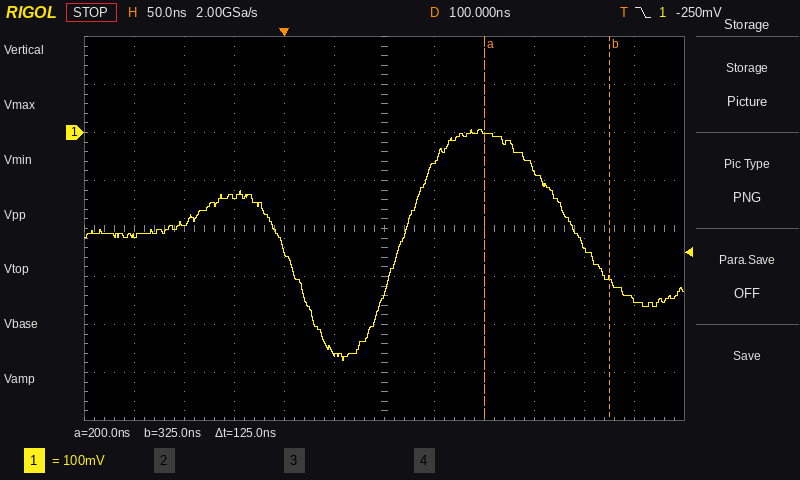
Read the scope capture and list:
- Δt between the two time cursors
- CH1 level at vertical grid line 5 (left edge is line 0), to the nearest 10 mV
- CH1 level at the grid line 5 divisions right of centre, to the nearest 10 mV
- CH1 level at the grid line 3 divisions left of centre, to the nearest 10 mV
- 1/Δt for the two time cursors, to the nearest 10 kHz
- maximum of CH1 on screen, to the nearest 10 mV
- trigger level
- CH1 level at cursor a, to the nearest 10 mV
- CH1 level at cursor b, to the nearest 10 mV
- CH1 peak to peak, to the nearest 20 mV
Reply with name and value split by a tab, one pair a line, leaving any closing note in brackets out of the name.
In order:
Δt between the two time cursors	125 ns
CH1 level at vertical grid line 5 (left edge is line 0), to the nearest 10 mV	-460 mV
CH1 level at the grid line 5 divisions right of centre, to the nearest 10 mV	-350 mV
CH1 level at the grid line 3 divisions left of centre, to the nearest 10 mV	-130 mV
1/Δt for the two time cursors, to the nearest 10 kHz	8.00 MHz
maximum of CH1 on screen, to the nearest 10 mV	10 mV
trigger level	-250 mV
CH1 level at cursor a, to the nearest 10 mV	0 mV
CH1 level at cursor b, to the nearest 10 mV	-310 mV
CH1 peak to peak, to the nearest 20 mV	480 mV
